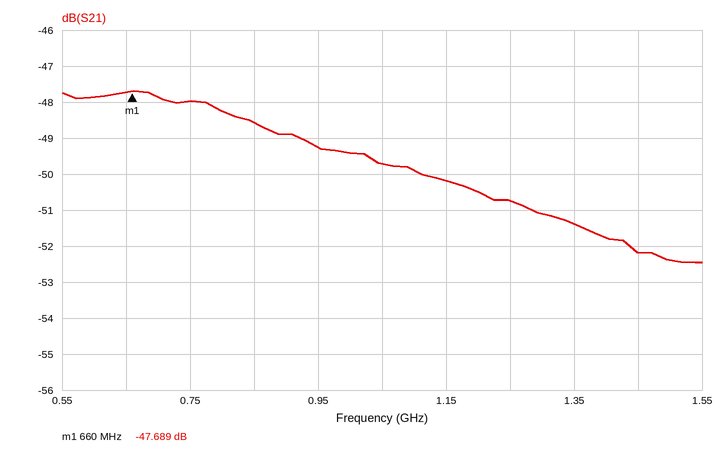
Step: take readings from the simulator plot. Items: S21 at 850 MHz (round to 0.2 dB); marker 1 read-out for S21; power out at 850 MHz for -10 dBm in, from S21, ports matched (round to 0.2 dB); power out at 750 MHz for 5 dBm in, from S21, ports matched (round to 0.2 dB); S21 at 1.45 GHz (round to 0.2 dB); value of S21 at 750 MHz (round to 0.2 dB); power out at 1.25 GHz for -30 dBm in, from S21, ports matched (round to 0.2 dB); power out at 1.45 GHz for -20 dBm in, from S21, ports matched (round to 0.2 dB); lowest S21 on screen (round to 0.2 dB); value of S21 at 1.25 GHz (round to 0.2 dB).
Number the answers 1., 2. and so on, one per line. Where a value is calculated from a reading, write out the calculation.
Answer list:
1. -48.6 dB
2. -47.689 dB
3. -10 dBm + (-48.6 dB) = -58.6 dBm
4. 5 dBm + (-48.0 dB) = -43.0 dBm
5. -52.2 dB
6. -48.0 dB
7. -30 dBm + (-50.8 dB) = -80.8 dBm
8. -20 dBm + (-52.2 dB) = -72.2 dBm
9. -52.4 dB
10. -50.8 dB
